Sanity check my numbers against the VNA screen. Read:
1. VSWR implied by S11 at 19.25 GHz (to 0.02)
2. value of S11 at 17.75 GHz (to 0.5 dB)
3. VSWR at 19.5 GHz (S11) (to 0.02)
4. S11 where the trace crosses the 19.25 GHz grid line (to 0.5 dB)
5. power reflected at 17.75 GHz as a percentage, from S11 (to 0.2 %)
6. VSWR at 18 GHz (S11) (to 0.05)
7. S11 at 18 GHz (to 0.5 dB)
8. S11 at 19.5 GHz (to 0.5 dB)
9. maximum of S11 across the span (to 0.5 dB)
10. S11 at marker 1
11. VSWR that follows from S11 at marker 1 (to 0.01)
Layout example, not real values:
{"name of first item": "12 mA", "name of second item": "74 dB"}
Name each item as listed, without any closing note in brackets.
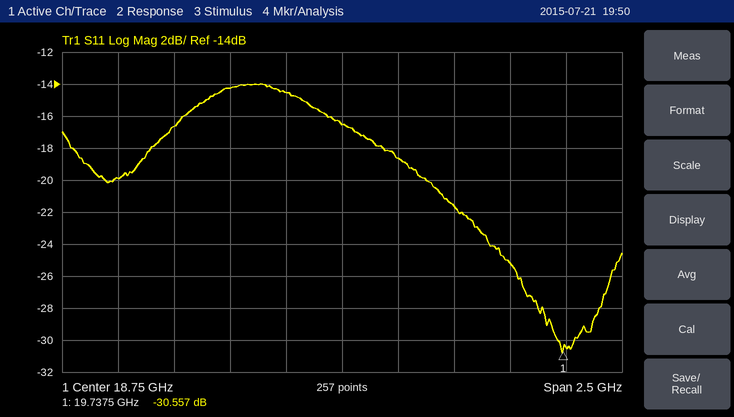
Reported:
{"VSWR implied by S11 at 19.25 GHz": "1.18", "value of S11 at 17.75 GHz": "-20.0 dB", "VSWR at 19.5 GHz (S11)": "1.12", "S11 where the trace crosses the 19.25 GHz grid line": "-21.5 dB", "power reflected at 17.75 GHz as a percentage, from S11": "1.0 %", "VSWR at 18 GHz (S11)": "1.35", "S11 at 18 GHz": "-16.5 dB", "S11 at 19.5 GHz": "-25.0 dB", "maximum of S11 across the span": "-14.0 dB", "S11 at marker 1": "-30.557 dB", "VSWR that follows from S11 at marker 1": "1.06"}
